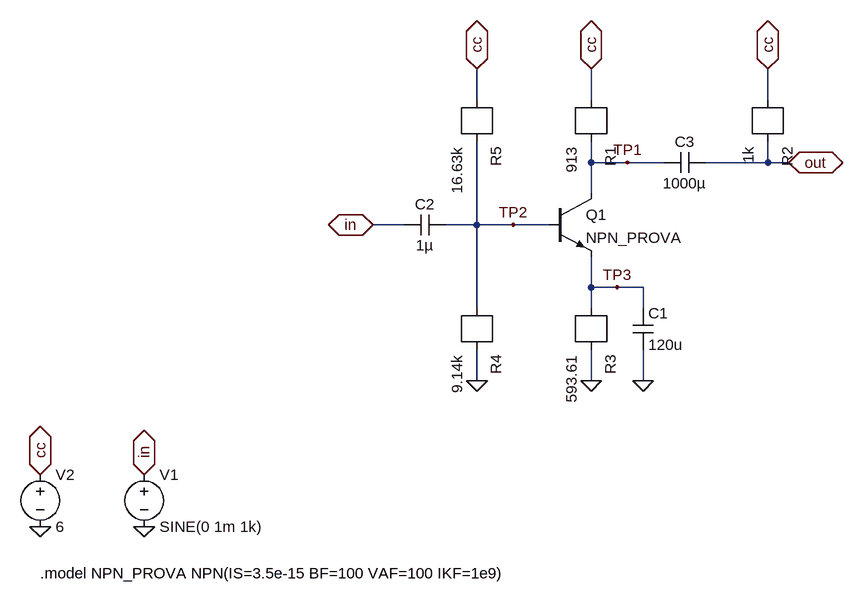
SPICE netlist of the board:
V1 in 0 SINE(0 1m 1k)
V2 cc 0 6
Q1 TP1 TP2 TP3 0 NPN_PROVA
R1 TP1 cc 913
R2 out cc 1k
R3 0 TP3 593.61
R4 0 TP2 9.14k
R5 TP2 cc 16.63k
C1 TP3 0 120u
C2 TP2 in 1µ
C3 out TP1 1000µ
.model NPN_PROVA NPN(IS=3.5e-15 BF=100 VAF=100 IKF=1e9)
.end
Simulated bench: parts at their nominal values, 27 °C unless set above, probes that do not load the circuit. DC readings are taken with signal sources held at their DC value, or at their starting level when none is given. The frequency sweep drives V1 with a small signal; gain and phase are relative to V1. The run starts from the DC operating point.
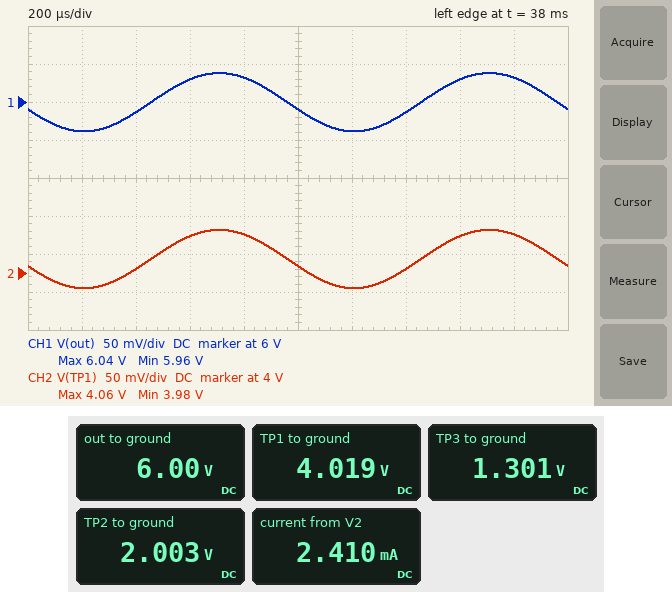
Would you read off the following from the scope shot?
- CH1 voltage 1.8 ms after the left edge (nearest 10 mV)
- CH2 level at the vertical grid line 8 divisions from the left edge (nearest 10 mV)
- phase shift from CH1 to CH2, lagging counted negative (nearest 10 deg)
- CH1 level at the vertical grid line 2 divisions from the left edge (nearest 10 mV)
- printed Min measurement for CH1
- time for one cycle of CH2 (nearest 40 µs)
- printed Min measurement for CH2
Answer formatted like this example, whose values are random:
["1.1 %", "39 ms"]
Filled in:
["6.03 V", "4.05 V", "0 deg", "5.99 V", "5.96 V", "1.00 ms", "3.98 V"]
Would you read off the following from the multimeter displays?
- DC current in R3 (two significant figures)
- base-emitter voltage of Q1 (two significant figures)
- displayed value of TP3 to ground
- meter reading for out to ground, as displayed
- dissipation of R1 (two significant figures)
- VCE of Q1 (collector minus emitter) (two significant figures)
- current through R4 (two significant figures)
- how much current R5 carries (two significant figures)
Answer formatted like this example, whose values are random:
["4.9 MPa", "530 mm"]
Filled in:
["2.2 mA", "700 mV", "1.301 V", "6.00 V", "4.3 mW", "2.7 V", "220 µA", "240 µA"]
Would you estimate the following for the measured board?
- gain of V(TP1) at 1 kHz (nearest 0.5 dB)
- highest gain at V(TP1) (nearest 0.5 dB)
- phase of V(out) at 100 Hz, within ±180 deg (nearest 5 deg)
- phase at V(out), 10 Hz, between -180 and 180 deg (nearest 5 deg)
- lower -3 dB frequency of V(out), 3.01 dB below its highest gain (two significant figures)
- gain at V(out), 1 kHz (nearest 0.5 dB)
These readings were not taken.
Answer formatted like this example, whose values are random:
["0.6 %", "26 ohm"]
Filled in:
["31.5 dB", "32.0 dB", "-105 deg", "-50 deg", "260 Hz", "31.5 dB"]
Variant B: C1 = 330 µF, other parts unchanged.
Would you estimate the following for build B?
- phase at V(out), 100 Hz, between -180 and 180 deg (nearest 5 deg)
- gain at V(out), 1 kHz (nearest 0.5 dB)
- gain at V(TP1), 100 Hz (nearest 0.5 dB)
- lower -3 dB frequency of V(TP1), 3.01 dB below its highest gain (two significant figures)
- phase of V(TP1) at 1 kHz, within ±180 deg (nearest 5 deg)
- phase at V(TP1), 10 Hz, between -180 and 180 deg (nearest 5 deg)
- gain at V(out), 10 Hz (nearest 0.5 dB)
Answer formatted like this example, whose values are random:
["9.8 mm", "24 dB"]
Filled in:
["-115 deg", "32.0 dB", "25.0 dB", "190 Hz", "-170 deg", "-65 deg", "5.0 dB"]
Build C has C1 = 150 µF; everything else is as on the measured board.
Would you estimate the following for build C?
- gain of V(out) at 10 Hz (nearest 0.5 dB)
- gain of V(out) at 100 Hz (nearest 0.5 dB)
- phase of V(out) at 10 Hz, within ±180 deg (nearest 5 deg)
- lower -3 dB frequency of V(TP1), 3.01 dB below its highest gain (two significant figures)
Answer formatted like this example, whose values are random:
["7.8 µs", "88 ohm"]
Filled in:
["1.0 dB", "23.5 dB", "-55 deg", "240 Hz"]
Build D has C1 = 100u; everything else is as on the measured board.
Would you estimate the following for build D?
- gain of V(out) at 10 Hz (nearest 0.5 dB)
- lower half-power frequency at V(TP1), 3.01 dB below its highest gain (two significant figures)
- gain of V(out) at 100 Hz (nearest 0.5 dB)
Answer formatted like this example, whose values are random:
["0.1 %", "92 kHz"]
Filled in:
["-1.5 dB", "280 Hz", "22.5 dB"]
